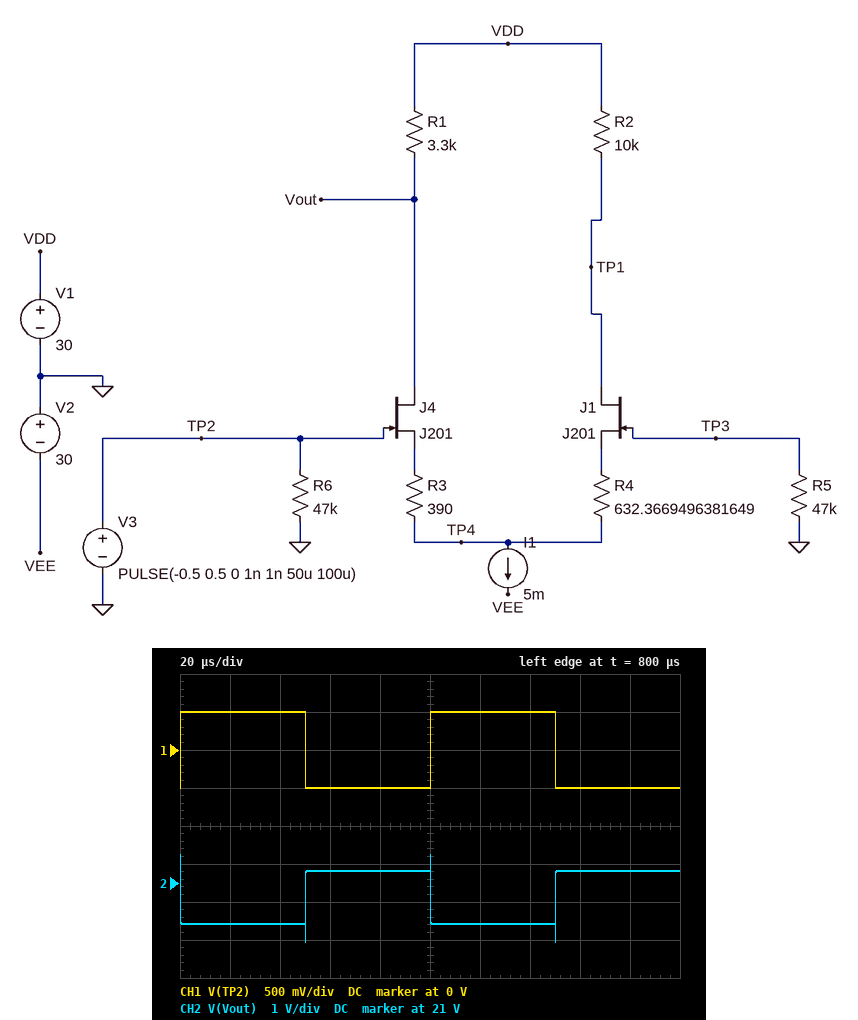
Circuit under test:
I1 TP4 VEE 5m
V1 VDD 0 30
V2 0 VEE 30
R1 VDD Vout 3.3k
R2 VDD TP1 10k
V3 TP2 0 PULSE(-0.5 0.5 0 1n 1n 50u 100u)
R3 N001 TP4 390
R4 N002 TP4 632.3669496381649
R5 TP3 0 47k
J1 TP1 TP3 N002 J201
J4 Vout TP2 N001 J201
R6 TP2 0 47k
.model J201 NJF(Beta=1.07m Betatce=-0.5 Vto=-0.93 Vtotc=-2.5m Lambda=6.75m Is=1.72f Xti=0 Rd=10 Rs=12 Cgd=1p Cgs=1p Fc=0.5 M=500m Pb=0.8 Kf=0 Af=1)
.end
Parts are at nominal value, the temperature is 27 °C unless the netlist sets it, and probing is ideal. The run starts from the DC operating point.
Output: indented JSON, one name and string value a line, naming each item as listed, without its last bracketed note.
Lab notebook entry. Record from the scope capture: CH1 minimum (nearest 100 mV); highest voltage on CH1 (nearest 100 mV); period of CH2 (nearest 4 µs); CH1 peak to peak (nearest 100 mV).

{
  "CH1 minimum": "-500 mV",
  "highest voltage on CH1": "500 mV",
  "period of CH2": "100 µs",
  "CH1 peak to peak": "1.0 V"
}
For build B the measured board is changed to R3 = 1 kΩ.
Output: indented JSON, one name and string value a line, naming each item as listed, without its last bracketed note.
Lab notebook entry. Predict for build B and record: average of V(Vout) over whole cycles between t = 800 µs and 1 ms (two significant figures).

{
  "average of V(Vout) over whole cycles between t = 800 µs and 1 ms": "22 V"
}
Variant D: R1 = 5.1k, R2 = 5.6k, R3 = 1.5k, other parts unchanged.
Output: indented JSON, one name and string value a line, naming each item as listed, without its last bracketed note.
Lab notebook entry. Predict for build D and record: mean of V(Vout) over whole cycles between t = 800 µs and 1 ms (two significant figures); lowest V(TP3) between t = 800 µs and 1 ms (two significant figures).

{
  "mean of V(Vout) over whole cycles between t = 800 µs and 1 ms": "19 V",
  "lowest V(TP3) between t = 800 µs and 1 ms": "-1.7 V"
}
